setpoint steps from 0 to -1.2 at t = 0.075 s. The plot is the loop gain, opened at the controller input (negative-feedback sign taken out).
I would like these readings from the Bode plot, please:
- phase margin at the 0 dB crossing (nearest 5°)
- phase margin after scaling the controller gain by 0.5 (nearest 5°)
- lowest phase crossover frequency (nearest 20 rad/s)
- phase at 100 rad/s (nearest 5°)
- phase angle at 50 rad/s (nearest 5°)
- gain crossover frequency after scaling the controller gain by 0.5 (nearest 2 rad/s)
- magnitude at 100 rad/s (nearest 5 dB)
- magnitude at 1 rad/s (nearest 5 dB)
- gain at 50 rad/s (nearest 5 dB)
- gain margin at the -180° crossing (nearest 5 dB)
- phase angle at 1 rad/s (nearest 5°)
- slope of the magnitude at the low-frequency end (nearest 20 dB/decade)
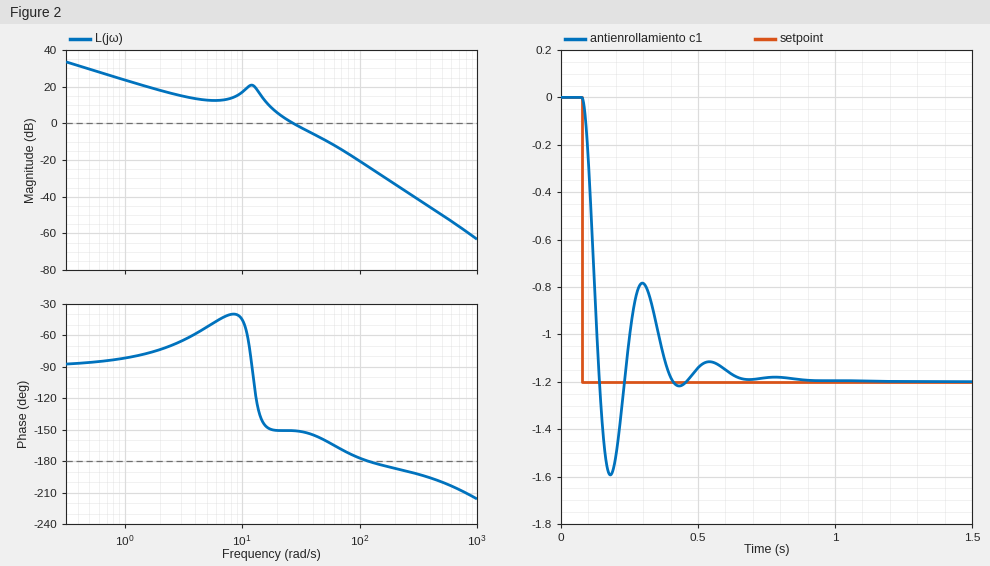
30°
30°
120 rad/s
-175°
-160°
20 rad/s
-20 dB
25 dB
-10 dB
25 dB
-80°
-20 dB/decade
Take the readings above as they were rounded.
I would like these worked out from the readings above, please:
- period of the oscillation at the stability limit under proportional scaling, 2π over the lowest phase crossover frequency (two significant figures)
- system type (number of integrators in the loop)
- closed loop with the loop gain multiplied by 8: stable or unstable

0.052 s
1
stable
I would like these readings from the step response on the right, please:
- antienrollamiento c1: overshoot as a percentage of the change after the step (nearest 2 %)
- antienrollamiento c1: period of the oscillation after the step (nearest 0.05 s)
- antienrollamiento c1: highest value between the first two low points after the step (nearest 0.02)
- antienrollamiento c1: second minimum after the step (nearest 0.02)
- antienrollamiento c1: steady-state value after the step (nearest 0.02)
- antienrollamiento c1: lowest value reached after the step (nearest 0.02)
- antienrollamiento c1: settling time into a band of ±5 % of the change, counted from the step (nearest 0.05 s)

32 %
0.25 s
-0.78
-1.22
-1.20
-1.60
0.50 s
